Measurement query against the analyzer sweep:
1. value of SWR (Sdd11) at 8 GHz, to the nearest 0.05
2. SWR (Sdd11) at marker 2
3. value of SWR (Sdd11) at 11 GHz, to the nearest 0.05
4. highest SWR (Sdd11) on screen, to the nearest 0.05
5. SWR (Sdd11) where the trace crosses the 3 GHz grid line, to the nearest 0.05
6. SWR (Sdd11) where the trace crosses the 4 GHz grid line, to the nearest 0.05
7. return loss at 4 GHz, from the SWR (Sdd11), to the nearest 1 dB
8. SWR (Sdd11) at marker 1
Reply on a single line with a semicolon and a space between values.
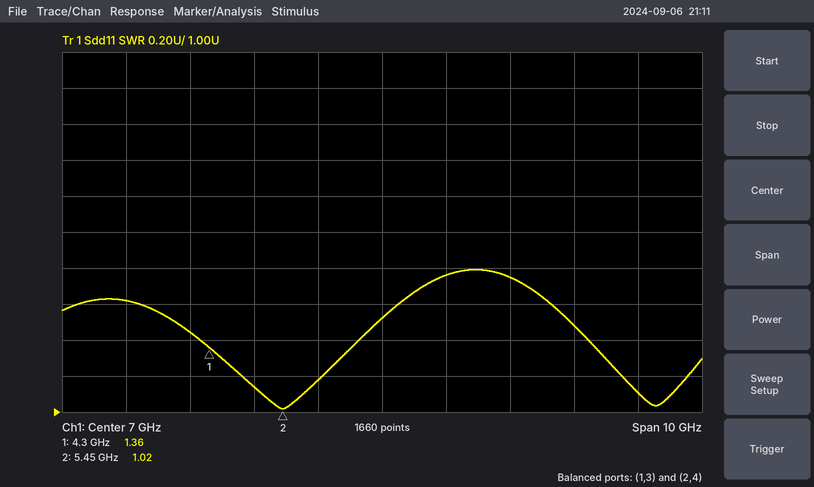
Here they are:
1.75; 1.02; 1.10; 1.80; 1.60; 1.45; 15 dB; 1.36
